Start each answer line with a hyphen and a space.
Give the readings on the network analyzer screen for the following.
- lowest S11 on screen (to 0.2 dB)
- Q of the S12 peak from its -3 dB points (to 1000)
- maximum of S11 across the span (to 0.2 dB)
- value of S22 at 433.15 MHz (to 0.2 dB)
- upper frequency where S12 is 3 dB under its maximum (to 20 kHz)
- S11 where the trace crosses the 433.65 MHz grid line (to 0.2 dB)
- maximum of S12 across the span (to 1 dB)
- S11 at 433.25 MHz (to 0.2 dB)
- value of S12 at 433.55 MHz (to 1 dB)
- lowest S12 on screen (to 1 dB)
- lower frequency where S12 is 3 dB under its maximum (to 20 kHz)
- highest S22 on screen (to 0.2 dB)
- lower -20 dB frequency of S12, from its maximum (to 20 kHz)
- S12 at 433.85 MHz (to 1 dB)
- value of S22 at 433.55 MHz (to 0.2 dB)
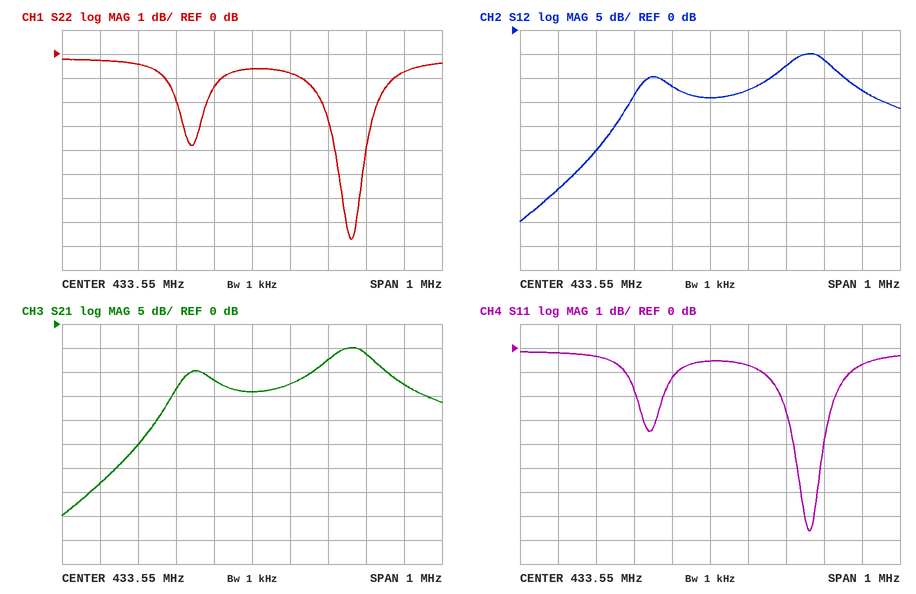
- -7.6 dB
- 3000
- -0.2 dB
- -0.2 dB
- 433.88 MHz
- -0.8 dB
- -5 dB
- -0.4 dB
- -14 dB
- -40 dB
- 433.74 MHz
- -0.2 dB
- 433.26 MHz
- -6 dB
- -0.6 dB
